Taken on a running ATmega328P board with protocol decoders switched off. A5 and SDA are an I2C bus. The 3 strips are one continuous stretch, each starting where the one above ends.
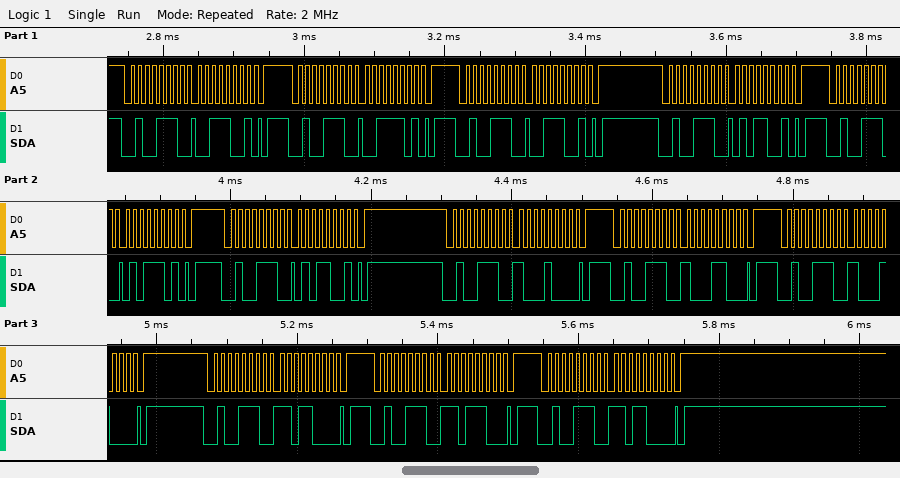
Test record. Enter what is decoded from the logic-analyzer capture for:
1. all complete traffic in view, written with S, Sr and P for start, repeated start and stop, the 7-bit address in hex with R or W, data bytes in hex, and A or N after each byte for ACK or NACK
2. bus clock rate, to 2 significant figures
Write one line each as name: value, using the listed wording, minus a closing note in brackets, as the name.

all complete traffic in view, written with S, Sr and P for start, repeated start and stop, the 7-bit address in hex with R or W, data bytes in hex, and A or N after each byte for ACK or NACK: S 27W A 39 A P S 27W A 3D A P S 27W A 39 A P S 27W A 59 A P S 27W A 5D A P S 27W A 59 A P S 27W A 88 A P S 27W A 8C A P S 27W A 88 A P S 27W A D8 A P S 27W A DC A P S 27W A D8 A P
bus clock rate, to 2 significant figures: 100 kHz
